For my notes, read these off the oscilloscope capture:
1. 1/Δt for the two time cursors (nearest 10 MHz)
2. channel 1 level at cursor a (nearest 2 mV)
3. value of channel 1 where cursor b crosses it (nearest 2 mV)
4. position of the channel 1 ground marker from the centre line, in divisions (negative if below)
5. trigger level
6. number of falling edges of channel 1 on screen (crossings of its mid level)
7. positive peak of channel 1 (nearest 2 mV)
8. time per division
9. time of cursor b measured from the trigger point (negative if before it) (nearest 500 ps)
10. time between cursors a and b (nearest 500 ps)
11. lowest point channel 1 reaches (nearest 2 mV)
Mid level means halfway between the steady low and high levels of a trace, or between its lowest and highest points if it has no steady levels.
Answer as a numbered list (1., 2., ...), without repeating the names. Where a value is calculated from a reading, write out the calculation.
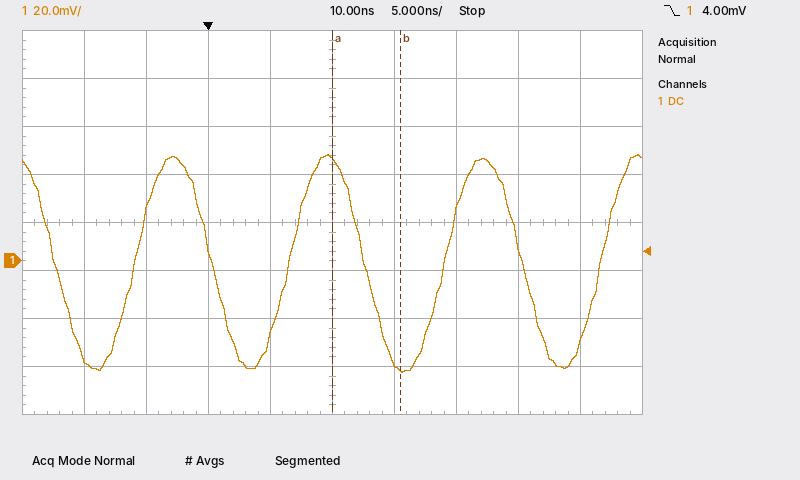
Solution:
1. 1 / 5.5 ns ≈ 180 MHz
2. 42 mV
3. -46 mV
4. -0.8 div
5. 4.00 mV
6. 4
7. 44 mV
8. 5 ns
9. +15.5 ns
10. 5.5 ns
11. -46 mV
